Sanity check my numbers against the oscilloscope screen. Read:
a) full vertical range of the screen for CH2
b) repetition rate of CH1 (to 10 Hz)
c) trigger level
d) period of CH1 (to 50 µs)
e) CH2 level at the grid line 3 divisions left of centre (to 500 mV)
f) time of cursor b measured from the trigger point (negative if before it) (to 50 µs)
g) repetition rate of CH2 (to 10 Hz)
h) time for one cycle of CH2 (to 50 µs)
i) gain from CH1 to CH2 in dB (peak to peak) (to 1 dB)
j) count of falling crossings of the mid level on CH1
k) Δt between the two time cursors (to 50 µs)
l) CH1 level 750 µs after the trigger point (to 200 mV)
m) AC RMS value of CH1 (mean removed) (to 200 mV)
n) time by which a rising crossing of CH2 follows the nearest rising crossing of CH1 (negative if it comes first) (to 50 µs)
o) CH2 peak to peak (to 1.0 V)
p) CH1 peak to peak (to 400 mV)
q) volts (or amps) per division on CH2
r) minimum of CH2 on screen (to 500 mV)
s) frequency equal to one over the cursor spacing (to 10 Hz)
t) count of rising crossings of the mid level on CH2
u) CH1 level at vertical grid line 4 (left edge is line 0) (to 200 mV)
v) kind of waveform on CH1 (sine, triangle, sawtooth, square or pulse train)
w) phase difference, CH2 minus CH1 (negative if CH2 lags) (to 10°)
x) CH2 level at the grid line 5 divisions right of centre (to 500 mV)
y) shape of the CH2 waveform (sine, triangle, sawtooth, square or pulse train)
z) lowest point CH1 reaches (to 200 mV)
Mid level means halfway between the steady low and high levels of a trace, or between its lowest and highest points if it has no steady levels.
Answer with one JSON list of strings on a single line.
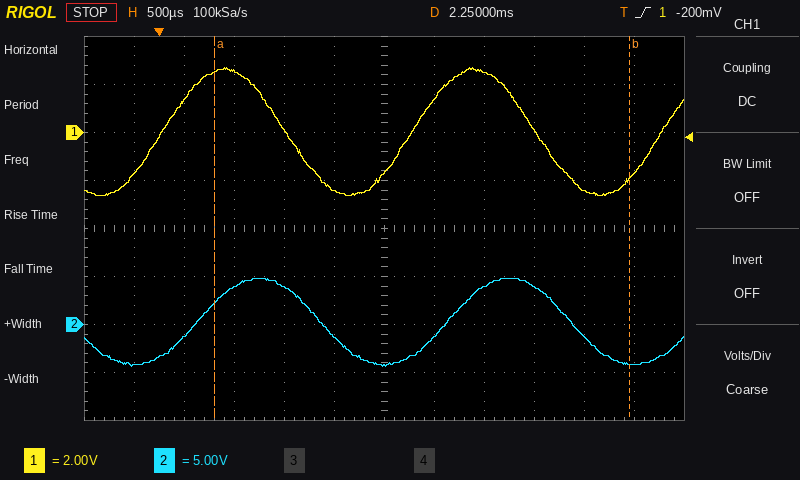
["40 V", "400 Hz", "-200 mV", "2.50 ms", "4.0 V", "+4.70 ms", "400 Hz", "2.50 ms", "5 dB", "2", "4.15 ms", "2.6 V", "1.8 V", "+350 µs", "9.0 V", "5.2 V", "5 V", "-4.5 V", "240 Hz", "2", "200 mV", "sine", "-50°", "-4.0 V", "sine", "-2.6 V"]
